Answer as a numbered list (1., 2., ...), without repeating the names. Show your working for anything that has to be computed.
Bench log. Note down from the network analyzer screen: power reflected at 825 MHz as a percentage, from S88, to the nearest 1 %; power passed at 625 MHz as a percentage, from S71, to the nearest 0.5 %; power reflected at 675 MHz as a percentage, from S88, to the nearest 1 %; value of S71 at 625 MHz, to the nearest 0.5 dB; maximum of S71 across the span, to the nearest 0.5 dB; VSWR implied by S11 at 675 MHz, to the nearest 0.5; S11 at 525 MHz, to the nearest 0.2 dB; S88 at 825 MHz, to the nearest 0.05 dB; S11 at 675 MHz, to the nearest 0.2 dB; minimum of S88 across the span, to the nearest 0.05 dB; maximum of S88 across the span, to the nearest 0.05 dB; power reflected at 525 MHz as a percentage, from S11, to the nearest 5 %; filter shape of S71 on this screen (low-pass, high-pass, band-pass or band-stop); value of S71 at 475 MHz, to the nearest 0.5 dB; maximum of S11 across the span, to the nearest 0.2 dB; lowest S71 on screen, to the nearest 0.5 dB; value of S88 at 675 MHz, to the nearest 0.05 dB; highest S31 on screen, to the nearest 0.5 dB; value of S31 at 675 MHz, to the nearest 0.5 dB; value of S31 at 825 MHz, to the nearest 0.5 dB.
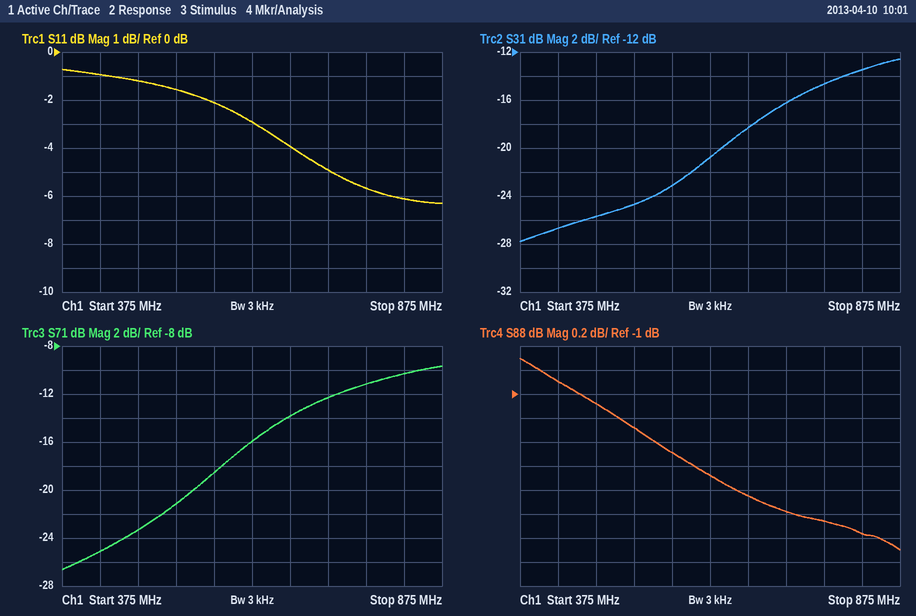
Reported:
1. 10^(-2.15/10) ≈ 61 %
2. 10^(-16/10) ≈ 2.5 %
3. 10^(-1.85/10) ≈ 65 %
4. -16.0 dB
5. -9.5 dB
6. |Γ| = 10^(-4/20) = 0.6310; VSWR = (1 + 0.6310)/(1 − 0.6310) ≈ 4.42, so 4.5 to the nearest 0.5
7. -1.6 dB
8. -2.15 dB
9. -4.0 dB
10. -2.30 dB
11. -0.70 dB
12. 10^(-1.6/10) ≈ 69.2 %, so 70 % to the nearest 5 %
13. high-pass
14. -23.5 dB
15. -0.8 dB
16. -26.5 dB
17. -1.85 dB
18. -12.5 dB
19. -18.5 dB
20. -13.5 dB
